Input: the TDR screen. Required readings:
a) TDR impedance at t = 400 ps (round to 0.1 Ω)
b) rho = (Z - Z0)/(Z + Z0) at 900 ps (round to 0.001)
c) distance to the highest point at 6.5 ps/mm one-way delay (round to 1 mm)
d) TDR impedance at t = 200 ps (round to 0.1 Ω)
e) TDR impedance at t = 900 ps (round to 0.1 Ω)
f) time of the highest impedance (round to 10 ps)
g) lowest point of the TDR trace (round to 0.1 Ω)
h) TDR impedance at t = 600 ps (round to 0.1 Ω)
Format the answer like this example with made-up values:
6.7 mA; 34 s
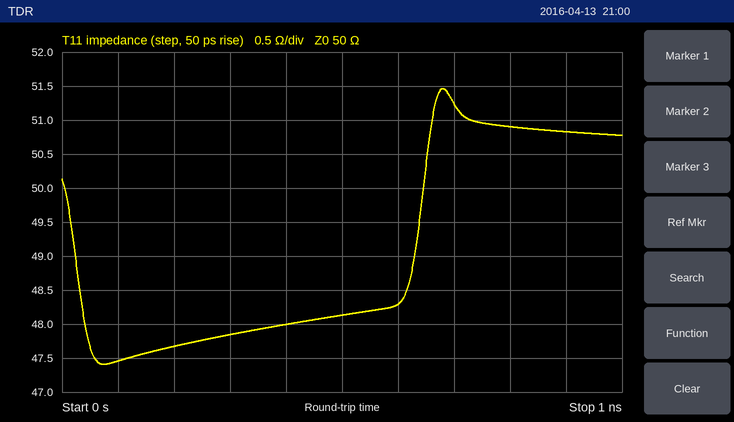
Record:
48.0 Ω; +0.008; 52 mm; 47.7 Ω; 50.8 Ω; 680 ps; 47.4 Ω; 48.3 Ω
